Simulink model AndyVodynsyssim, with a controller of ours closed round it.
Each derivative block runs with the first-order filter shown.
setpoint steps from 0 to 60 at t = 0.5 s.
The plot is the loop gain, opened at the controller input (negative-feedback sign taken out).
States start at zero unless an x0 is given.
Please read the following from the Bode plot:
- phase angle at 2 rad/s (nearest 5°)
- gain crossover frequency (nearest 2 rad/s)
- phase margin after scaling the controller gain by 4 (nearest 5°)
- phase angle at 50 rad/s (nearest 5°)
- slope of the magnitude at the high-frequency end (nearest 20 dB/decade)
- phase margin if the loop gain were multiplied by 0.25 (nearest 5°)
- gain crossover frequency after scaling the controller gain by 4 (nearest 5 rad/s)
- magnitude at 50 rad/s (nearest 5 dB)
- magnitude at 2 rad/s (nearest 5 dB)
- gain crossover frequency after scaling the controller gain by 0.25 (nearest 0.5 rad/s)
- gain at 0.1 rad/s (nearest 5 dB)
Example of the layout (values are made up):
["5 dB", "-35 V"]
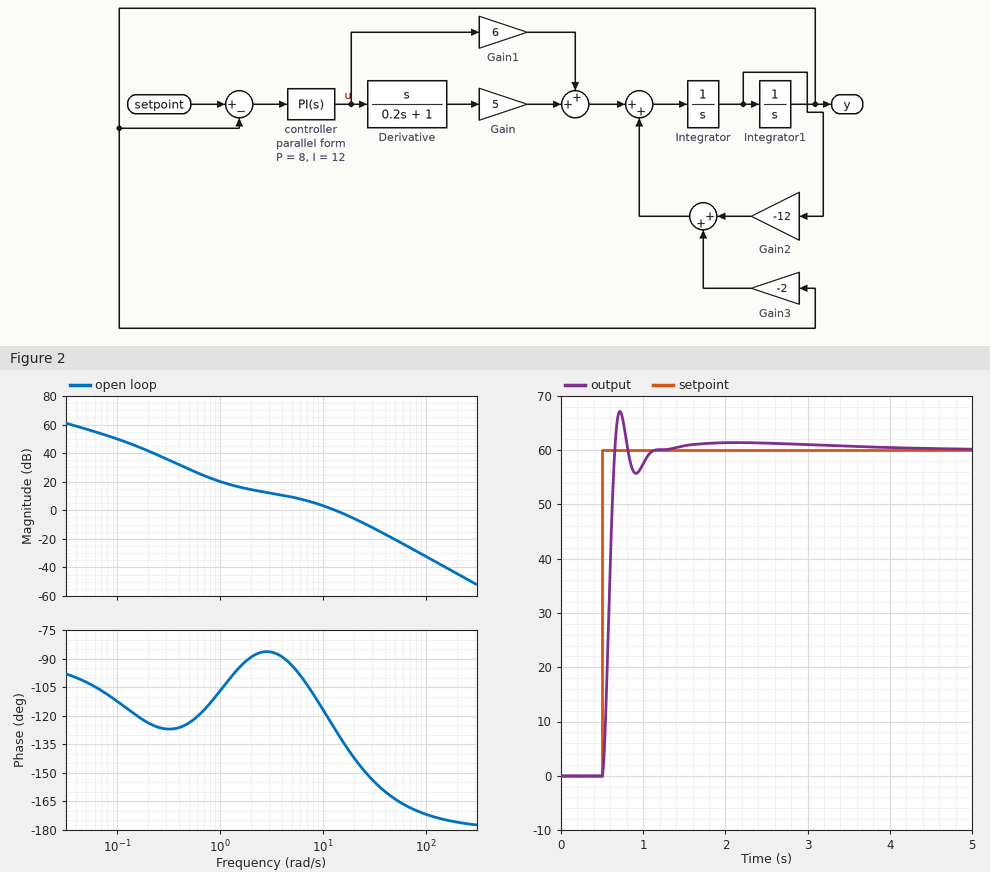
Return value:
["-90°", "14 rad/s", "25°", "-165°", "-40 dB/decade", "95°", "30 rad/s", "-20 dB", "15 dB", "3.0 rad/s", "50 dB"]
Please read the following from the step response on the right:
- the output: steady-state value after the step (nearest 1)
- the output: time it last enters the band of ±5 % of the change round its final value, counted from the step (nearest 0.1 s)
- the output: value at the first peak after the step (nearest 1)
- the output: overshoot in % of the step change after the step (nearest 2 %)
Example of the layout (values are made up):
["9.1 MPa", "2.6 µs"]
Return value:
["60", "0.5 s", "67", "12 %"]
